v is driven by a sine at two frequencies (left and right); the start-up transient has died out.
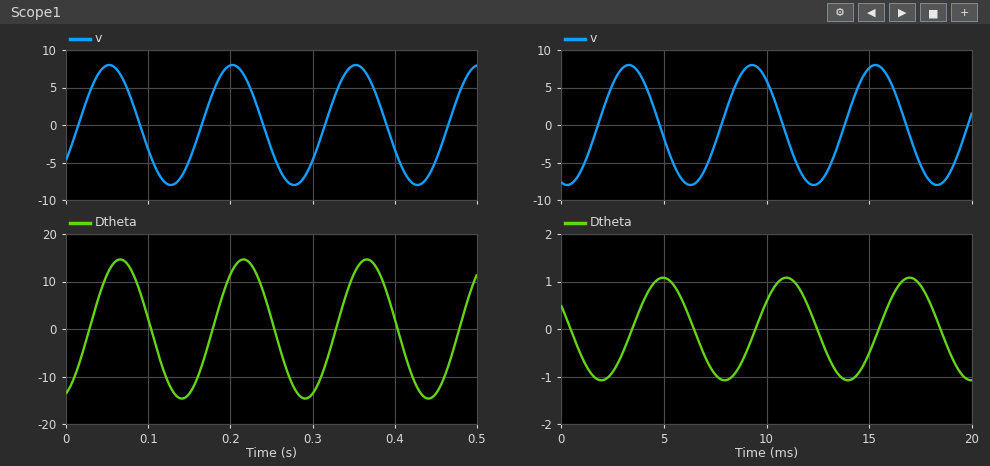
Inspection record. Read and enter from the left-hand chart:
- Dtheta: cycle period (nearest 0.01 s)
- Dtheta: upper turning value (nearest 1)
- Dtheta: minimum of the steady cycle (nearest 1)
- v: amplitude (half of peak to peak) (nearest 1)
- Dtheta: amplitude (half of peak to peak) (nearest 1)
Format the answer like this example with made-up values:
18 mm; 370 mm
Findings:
0.15 s; 15; -15; 8; 15
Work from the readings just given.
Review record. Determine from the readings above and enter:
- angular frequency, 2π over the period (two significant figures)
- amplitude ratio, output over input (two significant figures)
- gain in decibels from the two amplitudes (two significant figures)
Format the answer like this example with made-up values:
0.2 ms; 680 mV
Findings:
42 rad/s; 1.9; 5.5 dB
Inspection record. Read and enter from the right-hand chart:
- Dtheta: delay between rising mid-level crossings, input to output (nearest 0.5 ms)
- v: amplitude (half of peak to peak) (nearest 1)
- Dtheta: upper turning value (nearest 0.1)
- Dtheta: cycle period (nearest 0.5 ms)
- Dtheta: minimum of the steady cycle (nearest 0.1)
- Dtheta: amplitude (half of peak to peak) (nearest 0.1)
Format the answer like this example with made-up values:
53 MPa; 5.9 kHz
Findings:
1.5 ms; 8; 1.1; 6.0 ms; -1.1; 1.1
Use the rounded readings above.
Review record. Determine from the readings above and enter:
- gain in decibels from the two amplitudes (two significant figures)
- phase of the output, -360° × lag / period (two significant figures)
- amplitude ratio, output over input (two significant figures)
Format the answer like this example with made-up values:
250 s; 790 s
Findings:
-17 dB; -90°; 0.14
